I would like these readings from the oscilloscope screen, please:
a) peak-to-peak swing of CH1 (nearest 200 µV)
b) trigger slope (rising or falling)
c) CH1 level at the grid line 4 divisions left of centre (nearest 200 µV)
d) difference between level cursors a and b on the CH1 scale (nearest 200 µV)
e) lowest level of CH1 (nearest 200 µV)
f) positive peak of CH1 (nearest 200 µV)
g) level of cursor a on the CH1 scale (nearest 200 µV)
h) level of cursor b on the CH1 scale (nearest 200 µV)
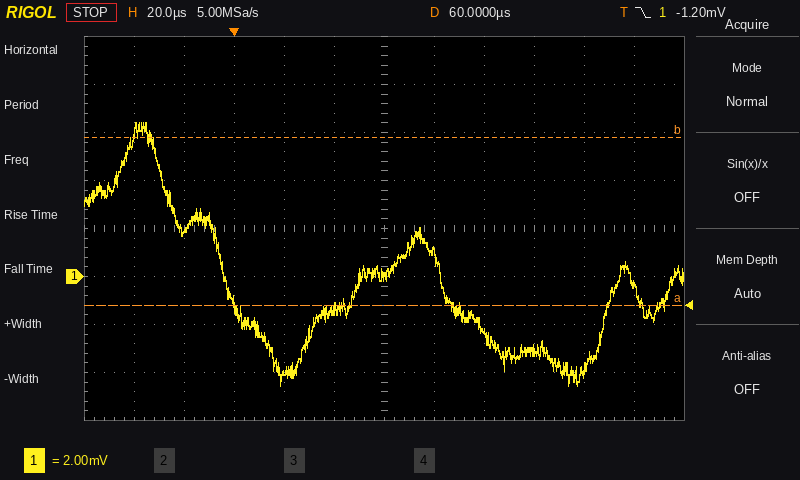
11.0 mV
falling
1.8 mV
7.0 mV
-4.6 mV
6.4 mV
-1.2 mV
5.8 mV
